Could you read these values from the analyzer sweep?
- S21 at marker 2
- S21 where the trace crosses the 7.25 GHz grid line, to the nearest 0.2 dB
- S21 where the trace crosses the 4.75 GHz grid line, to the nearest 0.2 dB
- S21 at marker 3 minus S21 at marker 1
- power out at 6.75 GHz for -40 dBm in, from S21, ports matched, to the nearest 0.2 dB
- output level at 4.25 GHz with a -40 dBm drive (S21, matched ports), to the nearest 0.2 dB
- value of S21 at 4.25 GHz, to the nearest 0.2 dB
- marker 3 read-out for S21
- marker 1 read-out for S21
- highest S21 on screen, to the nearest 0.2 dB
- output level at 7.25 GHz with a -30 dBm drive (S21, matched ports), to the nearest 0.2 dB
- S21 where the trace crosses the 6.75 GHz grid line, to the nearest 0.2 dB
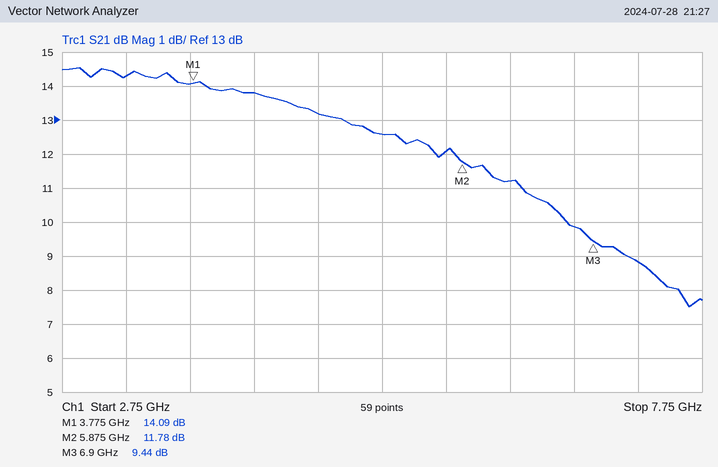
11.78 dB
8.8 dB
13.2 dB
-4.65 dB
-30.2 dBm
-26.2 dBm
13.8 dB
9.44 dB
14.09 dB
14.6 dB
-21.2 dBm
9.8 dB
